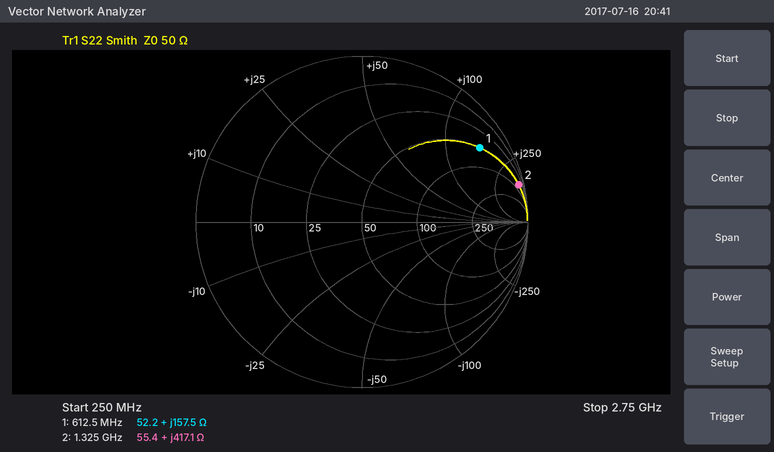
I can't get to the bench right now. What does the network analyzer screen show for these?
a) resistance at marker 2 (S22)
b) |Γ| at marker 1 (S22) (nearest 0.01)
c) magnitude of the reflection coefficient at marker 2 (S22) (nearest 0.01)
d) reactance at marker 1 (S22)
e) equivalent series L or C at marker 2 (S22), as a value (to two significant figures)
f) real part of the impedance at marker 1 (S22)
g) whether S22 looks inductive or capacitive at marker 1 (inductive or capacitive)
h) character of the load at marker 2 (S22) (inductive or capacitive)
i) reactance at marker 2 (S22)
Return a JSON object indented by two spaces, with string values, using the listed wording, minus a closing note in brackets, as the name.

{
  "resistance at marker 2": "55.4 Ω",
  "|Γ| at marker 1 (S22)": "0.84",
  "magnitude of the reflection coefficient at marker 2 (S22)": "0.97",
  "reactance at marker 1": "+157.5 Ω",
  "equivalent series L or C at marker 2 (S22), as a value": "50 nH",
  "real part of the impedance at marker 1": "52.2 Ω",
  "whether S22 looks inductive or capacitive at marker 1": "inductive",
  "character of the load at marker 2 (S22)": "inductive",
  "reactance at marker 2": "+417.1 Ω"
}
